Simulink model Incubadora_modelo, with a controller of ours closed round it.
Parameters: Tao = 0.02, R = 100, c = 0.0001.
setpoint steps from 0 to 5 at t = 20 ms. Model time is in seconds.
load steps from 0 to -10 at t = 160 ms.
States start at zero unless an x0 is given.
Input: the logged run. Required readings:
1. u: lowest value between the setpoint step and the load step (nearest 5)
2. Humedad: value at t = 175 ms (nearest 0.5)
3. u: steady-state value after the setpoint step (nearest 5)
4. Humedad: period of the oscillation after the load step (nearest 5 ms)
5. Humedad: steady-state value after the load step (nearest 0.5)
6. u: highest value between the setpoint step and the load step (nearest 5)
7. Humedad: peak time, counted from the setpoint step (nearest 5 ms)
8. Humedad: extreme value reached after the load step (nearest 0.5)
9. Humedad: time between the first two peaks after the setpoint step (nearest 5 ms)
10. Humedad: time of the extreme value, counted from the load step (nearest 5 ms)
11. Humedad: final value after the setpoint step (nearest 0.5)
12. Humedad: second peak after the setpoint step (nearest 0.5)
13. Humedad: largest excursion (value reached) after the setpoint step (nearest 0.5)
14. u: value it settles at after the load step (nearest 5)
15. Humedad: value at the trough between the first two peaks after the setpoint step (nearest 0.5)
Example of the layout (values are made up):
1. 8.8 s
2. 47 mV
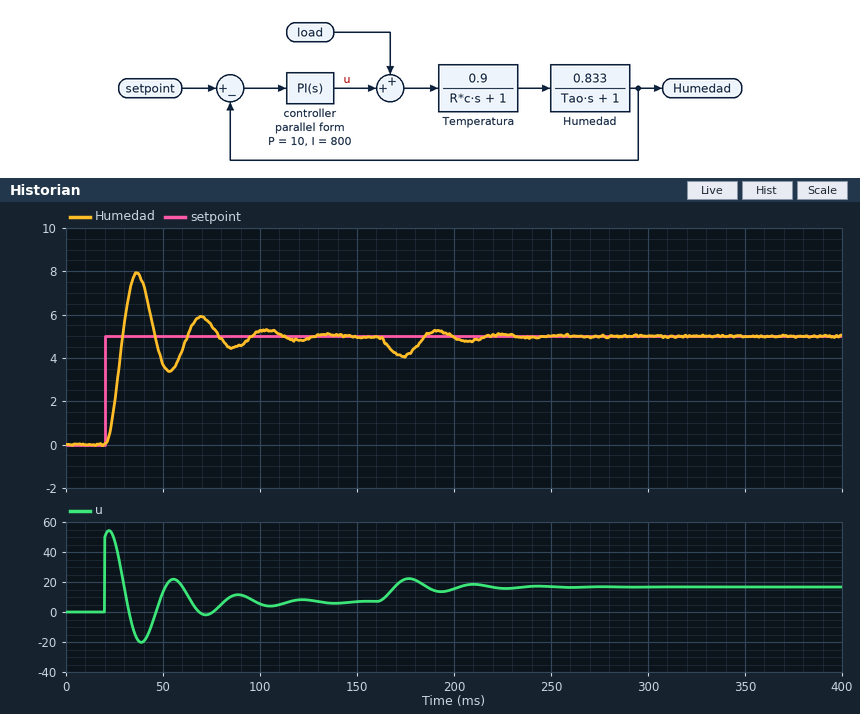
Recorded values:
1. -20
2. 4.0
3. 5
4. 35 ms
5. 5.0
6. 55
7. 15 ms
8. 4.0
9. 35 ms
10. 15 ms
11. 5.0
12. 6.0
13. 8.0
14. 15
15. 3.5
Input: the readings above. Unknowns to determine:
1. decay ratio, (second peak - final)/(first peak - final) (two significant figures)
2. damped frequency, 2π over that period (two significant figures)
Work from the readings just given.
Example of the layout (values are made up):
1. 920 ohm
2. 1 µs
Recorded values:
1. 0.33
2. 0.18 rad/ms
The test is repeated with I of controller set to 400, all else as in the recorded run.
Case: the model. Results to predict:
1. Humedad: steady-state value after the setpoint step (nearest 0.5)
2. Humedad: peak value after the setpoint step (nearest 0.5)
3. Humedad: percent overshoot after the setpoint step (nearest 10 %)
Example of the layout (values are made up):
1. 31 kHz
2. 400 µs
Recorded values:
1. 5.0
2. 7.0
3. 40 %
